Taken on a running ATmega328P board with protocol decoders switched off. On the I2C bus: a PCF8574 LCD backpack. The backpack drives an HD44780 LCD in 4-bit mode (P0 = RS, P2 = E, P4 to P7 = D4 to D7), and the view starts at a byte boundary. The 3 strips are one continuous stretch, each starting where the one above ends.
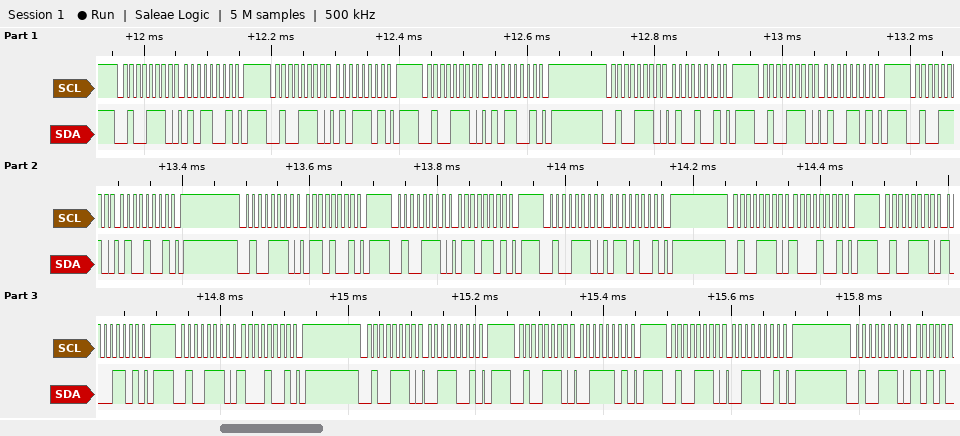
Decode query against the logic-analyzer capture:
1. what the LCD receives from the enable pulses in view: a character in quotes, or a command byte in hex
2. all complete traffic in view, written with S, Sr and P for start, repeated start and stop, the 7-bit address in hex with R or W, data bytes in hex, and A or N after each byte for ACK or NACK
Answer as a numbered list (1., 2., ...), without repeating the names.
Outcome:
1. 'T' 'h'
2. S 27W A 59 A P S 27W A 5D A P S 27W A 59 A P S 27W A 49 A P S 27W A 4D A P S 27W A 49 A P S 27W A 69 A P S 27W A 6D A P S 27W A 69 A P S 27W A 89 A P S 27W A 8D A P S 27W A 89 A P S 27W A 39 A P S 27W A 3D A P S 27W A 39 A P S 27W A
